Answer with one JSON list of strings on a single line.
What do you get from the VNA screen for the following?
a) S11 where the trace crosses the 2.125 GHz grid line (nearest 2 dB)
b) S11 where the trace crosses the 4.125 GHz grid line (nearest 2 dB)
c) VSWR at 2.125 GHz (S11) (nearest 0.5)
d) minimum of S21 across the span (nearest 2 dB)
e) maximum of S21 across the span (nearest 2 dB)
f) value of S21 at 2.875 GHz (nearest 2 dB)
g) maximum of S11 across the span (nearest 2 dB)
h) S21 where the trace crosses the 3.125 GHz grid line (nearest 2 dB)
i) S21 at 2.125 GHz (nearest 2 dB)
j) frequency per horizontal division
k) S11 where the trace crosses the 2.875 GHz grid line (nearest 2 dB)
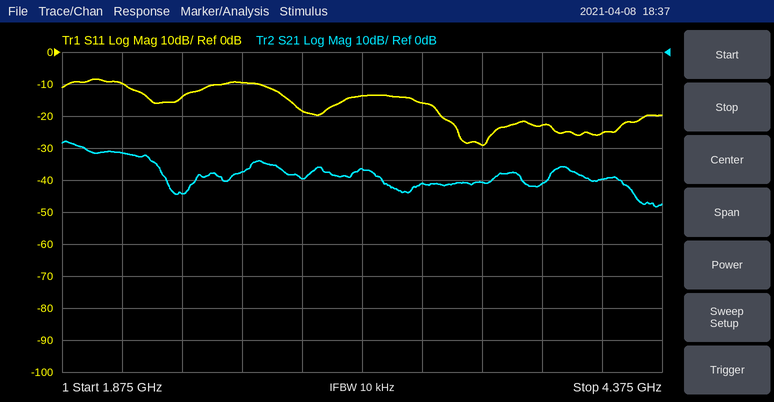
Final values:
["-10 dB", "-26 dB", "2.0", "-48 dB", "-28 dB", "-40 dB", "-8 dB", "-36 dB", "-32 dB", "250 MHz", "-18 dB"]
